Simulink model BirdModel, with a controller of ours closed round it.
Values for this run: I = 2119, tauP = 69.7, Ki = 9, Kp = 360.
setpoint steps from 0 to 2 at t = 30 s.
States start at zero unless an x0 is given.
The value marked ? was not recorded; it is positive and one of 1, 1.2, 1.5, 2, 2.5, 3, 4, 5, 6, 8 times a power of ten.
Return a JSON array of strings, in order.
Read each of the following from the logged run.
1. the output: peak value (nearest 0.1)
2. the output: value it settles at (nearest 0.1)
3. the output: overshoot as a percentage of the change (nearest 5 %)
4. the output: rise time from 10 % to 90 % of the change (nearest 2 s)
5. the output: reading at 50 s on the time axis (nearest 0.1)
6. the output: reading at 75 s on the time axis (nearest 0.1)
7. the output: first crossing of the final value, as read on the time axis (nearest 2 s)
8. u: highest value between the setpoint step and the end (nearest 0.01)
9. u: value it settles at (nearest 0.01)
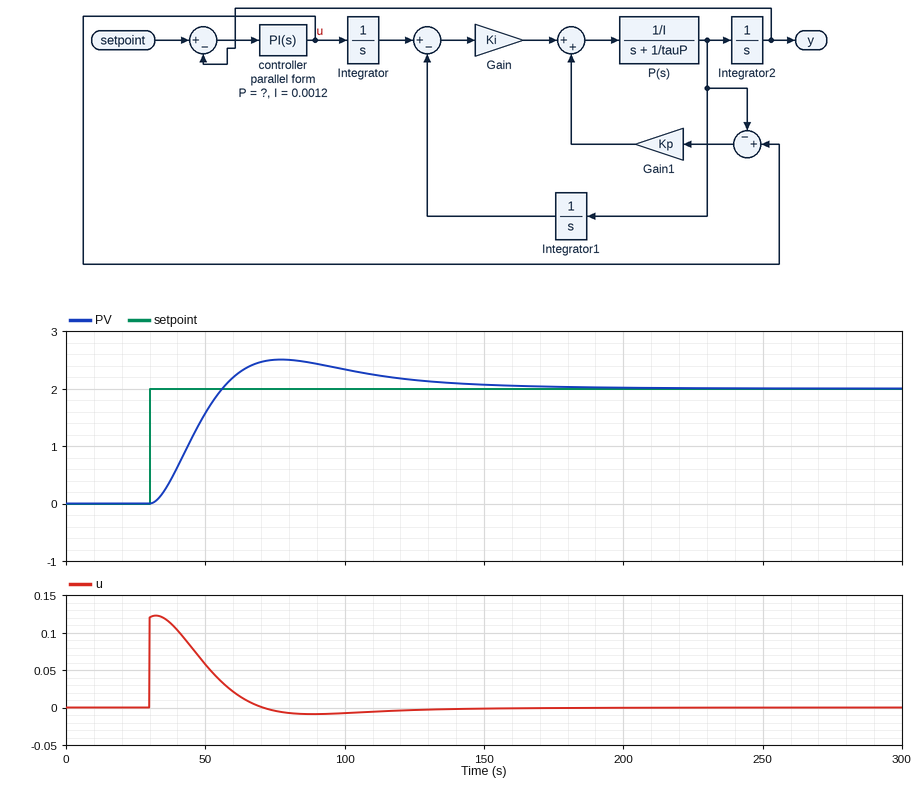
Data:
["2.5", "2.0", "25 %", "18 s", "1.6", "2.5", "56 s", "0.12", "0.00"]
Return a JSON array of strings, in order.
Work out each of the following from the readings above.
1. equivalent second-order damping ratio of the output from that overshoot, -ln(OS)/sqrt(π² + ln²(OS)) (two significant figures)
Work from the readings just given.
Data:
["0.40"]
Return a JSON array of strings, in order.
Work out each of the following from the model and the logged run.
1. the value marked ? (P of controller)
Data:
["0.06"]
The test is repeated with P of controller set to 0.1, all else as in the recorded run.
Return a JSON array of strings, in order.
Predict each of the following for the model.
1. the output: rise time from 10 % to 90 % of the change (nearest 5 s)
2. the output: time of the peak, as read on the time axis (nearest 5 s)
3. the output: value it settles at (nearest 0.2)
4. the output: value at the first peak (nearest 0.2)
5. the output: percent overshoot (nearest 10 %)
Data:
["15 s", "60 s", "2.0", "2.4", "20 %"]
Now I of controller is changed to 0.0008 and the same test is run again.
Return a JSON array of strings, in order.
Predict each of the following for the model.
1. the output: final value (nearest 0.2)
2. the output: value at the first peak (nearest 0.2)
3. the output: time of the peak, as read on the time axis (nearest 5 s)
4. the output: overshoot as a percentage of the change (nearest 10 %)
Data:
["2.0", "2.4", "80 s", "20 %"]
